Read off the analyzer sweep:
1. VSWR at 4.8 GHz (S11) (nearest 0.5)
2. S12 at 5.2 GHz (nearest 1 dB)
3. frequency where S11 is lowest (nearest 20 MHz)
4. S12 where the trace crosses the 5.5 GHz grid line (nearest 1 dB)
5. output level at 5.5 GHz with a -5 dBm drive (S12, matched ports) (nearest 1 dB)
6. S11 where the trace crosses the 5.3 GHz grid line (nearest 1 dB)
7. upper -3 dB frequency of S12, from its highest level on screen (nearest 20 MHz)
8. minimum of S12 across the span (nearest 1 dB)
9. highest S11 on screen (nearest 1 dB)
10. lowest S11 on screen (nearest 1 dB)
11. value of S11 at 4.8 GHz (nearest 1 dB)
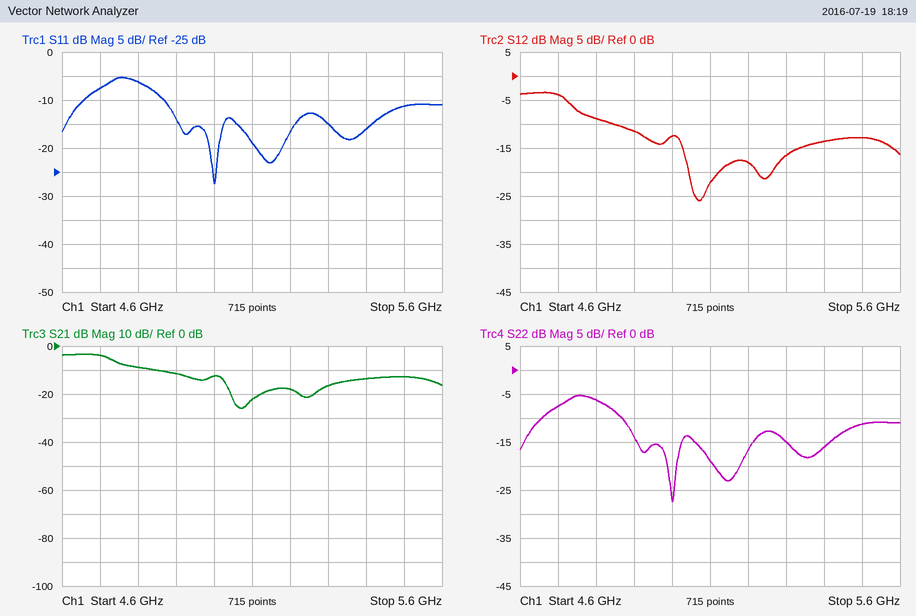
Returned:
3.0
-18 dB
5.00 GHz
-13 dB
-18 dBm
-15 dB
4.74 GHz
-26 dB
-5 dB
-27 dB
-6 dB
